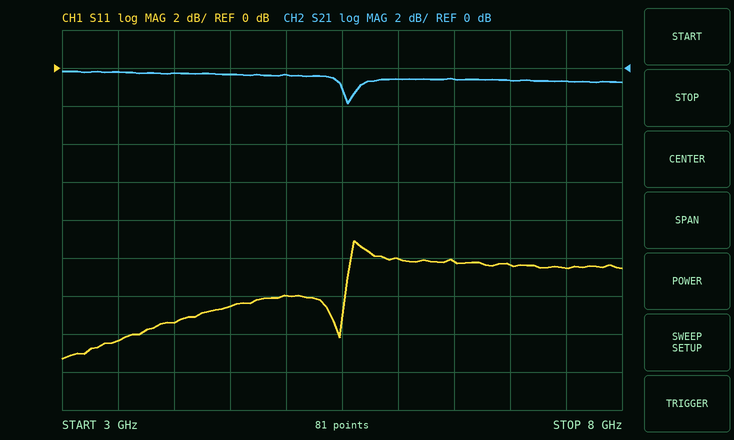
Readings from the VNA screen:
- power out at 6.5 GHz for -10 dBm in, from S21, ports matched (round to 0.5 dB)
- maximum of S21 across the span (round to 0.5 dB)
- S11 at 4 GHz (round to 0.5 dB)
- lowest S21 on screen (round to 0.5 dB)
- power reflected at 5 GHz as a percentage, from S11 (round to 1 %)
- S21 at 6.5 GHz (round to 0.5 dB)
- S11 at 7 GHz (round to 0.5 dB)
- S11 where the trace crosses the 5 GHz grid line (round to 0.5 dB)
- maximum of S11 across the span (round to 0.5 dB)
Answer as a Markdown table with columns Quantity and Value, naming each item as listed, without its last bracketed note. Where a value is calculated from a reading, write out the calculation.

| Quantity | Value |
|---|---|
| power out at 6.5 GHz for -10 dBm in, from S21, ports matched | -10 dBm + (-0.5 dB) = -10.5 dBm |
| maximum of S21 across the span | 0.0 dB |
| S11 at 4 GHz | -13.5 dB |
| lowest S21 on screen | -2.0 dB |
| power reflected at 5 GHz as a percentage, from S11 | 10^(-12/10) ≈ 6 % |
| S21 at 6.5 GHz | -0.5 dB |
| S11 at 7 GHz | -10.5 dB |
| S11 where the trace crosses the 5 GHz grid line | -12.0 dB |
| maximum of S11 across the span | -9.0 dB |
